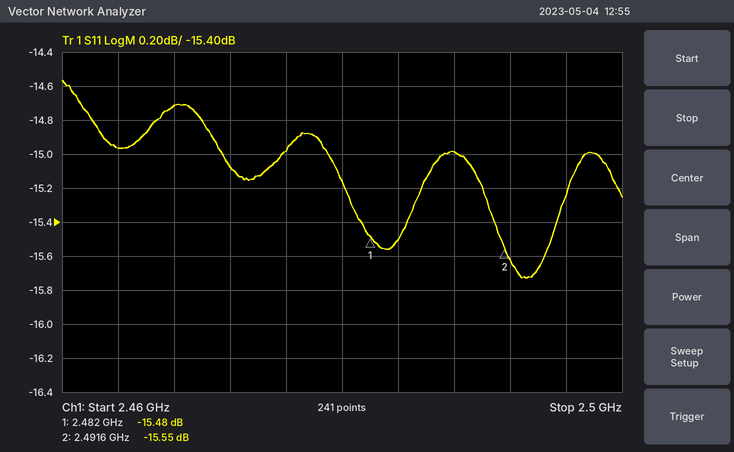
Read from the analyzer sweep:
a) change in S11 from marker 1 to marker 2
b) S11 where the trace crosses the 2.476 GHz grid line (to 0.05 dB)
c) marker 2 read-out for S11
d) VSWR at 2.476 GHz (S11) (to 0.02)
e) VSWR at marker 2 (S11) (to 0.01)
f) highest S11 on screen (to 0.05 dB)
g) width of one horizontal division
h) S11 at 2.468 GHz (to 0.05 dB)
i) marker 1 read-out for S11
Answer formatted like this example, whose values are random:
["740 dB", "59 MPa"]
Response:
["-0.07 dB", "-15.00 dB", "-15.55 dB", "1.44", "1.40", "-14.55 dB", "4 MHz", "-14.70 dB", "-15.48 dB"]
